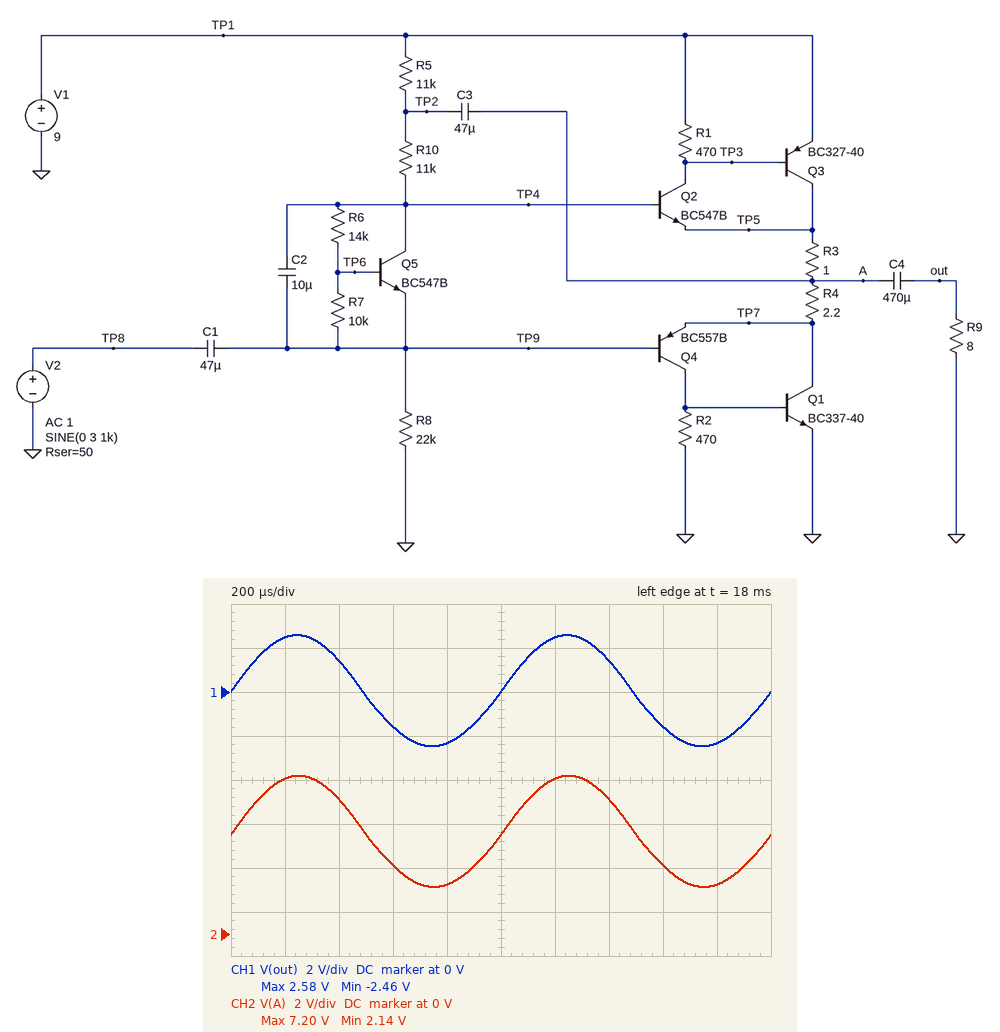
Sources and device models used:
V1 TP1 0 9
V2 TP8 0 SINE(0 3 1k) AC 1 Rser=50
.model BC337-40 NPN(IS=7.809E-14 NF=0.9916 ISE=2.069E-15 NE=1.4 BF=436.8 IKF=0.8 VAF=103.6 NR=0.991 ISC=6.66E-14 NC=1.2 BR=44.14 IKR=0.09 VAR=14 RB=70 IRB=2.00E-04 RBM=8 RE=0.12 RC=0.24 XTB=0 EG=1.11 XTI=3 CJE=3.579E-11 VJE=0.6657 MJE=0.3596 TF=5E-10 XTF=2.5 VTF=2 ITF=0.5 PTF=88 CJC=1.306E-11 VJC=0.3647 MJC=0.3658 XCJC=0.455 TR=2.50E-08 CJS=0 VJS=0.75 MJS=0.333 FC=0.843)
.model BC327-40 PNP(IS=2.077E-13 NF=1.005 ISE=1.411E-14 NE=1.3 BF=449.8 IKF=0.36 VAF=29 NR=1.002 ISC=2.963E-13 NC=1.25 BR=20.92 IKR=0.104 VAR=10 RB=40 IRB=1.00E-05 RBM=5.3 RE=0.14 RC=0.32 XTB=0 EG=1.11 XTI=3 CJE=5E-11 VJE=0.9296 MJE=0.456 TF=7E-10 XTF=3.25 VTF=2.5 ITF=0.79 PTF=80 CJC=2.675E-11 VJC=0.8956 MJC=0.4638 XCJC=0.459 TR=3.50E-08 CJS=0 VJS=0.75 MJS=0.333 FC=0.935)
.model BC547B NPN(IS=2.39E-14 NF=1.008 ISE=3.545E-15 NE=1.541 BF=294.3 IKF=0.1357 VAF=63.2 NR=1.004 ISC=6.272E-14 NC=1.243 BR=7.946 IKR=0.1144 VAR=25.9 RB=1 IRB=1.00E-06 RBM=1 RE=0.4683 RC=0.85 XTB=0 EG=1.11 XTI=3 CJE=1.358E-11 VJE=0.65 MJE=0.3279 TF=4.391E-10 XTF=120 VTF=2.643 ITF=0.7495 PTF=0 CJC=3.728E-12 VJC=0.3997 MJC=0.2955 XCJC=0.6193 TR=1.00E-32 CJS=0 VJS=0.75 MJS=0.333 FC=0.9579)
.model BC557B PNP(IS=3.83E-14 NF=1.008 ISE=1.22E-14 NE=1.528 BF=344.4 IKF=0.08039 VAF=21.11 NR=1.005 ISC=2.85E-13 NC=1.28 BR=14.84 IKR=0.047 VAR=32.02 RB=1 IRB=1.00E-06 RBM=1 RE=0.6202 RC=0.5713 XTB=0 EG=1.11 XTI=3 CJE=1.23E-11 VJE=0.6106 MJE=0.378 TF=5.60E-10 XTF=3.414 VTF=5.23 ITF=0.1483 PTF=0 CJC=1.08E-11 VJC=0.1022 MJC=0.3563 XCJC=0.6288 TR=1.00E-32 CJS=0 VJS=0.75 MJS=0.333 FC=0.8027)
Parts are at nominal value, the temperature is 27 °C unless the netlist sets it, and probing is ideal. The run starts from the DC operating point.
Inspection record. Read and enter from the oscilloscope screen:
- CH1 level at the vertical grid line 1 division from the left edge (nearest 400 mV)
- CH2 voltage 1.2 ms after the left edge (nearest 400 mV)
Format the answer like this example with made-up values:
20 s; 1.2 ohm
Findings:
2.4 V; 7.2 V
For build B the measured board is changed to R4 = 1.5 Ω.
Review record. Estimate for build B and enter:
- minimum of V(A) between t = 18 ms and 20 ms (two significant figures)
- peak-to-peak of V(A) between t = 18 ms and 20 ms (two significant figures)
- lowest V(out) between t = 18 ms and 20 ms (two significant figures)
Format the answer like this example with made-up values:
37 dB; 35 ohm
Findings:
1.9 V; 5.2 V; -2.6 V
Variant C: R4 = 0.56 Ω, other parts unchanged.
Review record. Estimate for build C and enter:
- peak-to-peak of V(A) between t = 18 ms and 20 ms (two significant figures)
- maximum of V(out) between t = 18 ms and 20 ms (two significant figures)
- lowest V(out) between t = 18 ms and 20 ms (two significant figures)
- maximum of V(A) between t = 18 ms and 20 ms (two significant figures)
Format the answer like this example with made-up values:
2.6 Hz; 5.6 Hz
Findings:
5.5 V; 2.7 V; -2.8 V; 7.2 V
